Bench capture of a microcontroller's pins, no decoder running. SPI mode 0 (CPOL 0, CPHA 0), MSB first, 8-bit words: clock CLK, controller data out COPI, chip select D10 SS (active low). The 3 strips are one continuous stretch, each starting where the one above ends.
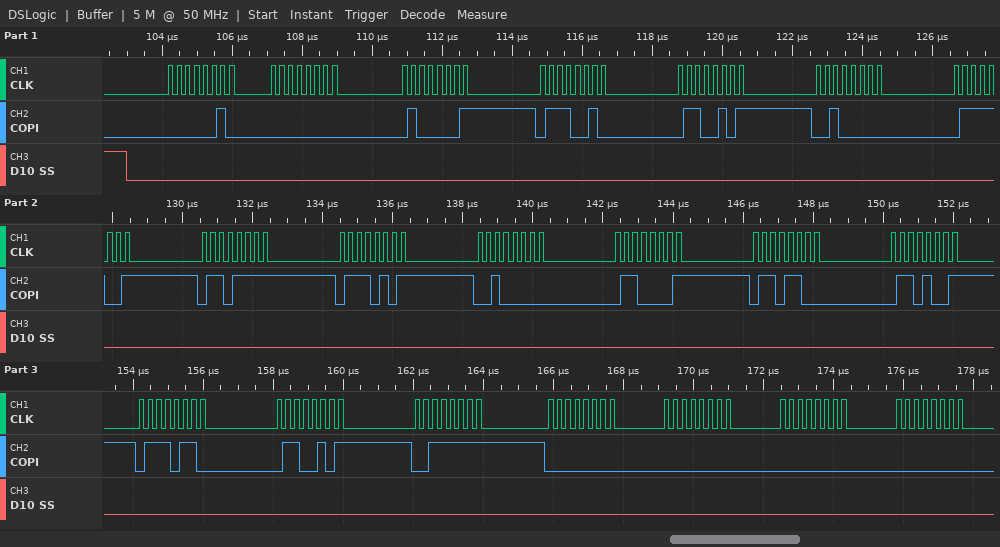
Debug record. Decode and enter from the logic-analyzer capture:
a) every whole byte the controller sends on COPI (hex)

02 00 41 72 65 20 79 6F 75 20 61 6C 69 76 65 3F 00 00 00 00
